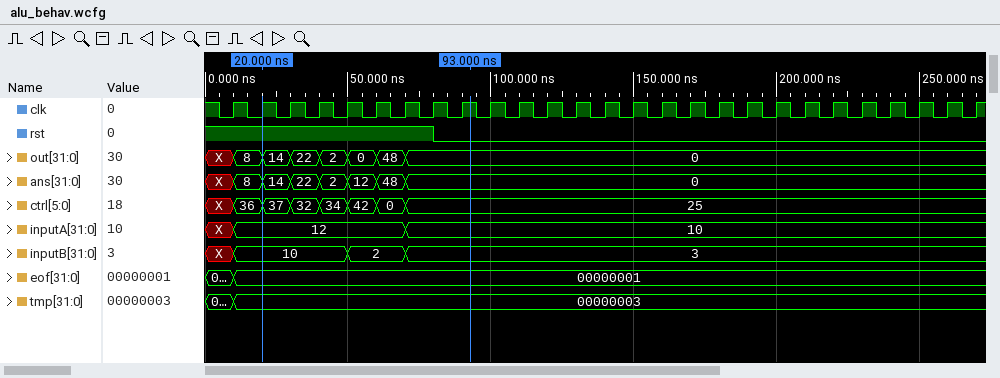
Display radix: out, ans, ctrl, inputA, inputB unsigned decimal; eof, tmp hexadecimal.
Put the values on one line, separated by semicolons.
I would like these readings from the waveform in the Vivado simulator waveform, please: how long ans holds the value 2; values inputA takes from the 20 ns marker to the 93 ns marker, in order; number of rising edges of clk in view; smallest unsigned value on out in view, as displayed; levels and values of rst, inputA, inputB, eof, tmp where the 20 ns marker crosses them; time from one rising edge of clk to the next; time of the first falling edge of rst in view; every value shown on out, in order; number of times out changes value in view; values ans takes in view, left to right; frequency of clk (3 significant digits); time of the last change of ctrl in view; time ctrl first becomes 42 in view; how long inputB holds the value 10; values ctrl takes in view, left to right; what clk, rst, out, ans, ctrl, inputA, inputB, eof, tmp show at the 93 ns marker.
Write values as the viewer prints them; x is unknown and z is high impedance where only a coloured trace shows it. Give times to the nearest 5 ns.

10 ns; 12, 10; 27; 0; rst=1, inputA=12, inputB=10, eof=00000001, tmp=00000003; 10 ns; 80 ns; X, 8, 14, 22, 2, 0, 48, 0; 7; X, 8, 14, 22, 2, 12, 48, 0; 100 MHz; 70 ns; 50 ns; 40 ns; X, 36, 37, 32, 34, 42, 0, 25; clk=1, rst=0, out=0, ans=0, ctrl=25, inputA=10, inputB=3, eof=00000001, tmp=00000003
